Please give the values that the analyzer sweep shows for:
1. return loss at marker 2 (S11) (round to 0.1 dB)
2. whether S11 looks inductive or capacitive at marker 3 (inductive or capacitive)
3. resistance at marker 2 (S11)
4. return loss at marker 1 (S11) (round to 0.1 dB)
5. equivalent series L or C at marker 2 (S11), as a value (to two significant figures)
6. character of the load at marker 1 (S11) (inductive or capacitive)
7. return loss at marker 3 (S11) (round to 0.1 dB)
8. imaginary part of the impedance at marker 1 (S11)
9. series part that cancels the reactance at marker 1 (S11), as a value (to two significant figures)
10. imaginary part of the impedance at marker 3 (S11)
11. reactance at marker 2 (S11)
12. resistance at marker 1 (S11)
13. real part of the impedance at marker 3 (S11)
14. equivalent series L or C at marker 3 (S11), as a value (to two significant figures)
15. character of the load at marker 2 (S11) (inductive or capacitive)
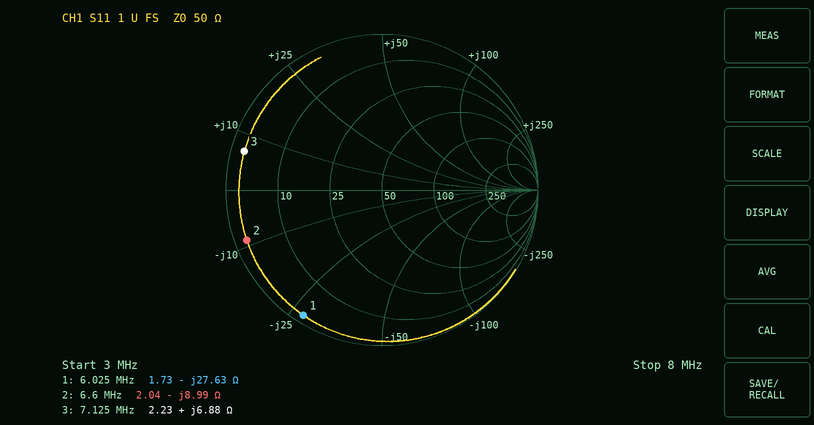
0.7 dB
inductive
2.04 Ω
0.5 dB
2.7 nF
capacitive
0.8 dB
-27.63 Ω
730 nH
+6.88 Ω
-8.99 Ω
1.73 Ω
2.23 Ω
150 nH
capacitive
